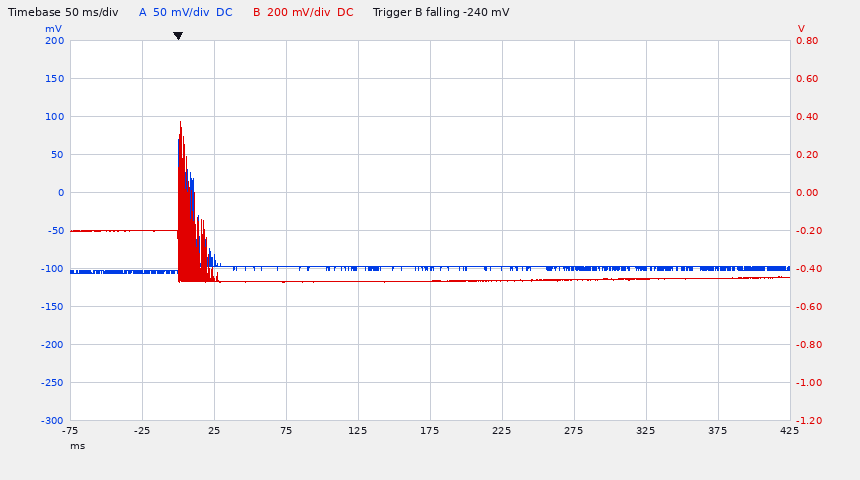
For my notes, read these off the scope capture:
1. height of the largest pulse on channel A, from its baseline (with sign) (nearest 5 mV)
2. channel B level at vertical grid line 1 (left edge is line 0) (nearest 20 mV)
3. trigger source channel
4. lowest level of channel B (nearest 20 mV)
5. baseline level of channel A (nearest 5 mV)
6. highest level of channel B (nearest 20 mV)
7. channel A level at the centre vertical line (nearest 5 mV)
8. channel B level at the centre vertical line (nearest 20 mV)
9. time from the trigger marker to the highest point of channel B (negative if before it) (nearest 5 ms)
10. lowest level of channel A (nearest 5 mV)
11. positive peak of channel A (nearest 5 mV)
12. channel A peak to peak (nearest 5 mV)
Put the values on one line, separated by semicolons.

+170 mV; -200 mV; channel B; -480 mV; -100 mV; 380 mV; -100 mV; -460 mV; 0 ms; -105 mV; 70 mV; 175 mV
